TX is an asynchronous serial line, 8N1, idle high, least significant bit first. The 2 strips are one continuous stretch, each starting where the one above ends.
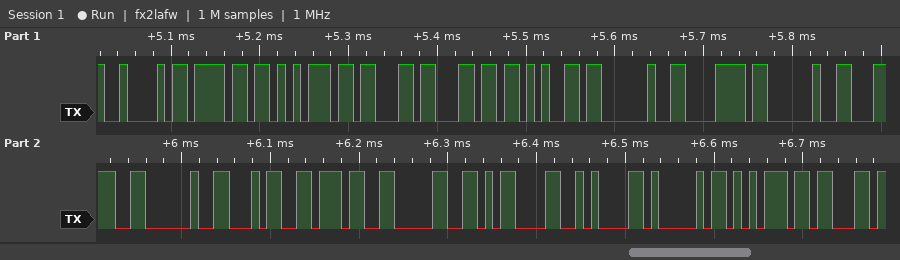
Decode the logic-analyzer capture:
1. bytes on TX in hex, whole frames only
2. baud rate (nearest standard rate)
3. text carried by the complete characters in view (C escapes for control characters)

42 6F 75 63 6C 65 20 78 20 3C 20 34 37 30 0D 0A 41 75 63
115200 baud
"Boucle x < 470\r\nAuc"
